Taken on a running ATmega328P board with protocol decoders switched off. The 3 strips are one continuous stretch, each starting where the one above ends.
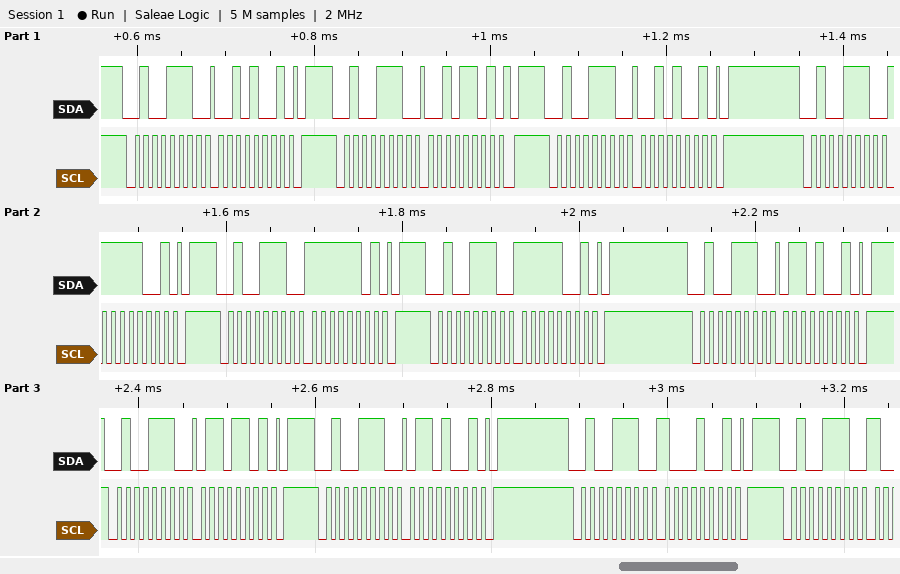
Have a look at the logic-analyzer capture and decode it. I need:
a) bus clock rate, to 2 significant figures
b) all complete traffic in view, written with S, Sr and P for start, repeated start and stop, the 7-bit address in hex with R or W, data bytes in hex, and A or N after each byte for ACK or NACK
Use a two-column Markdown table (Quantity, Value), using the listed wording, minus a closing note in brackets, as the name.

| Quantity | Value |
|---|---|
| bus clock rate, to 2 significant figures | 100 kHz |
| all complete traffic in view, written with S, Sr and P for start, repeated start and stop, the 7-bit address in hex with R or W, data bytes in hex, and A or N after each byte for ACK or NACK | S 27W A 29 A P S 27W A 2D A P S 27W A 29 A P S 27W A F9 A P S 27W A FD A P S 27W A F9 A P S 27W A 69 A P S 27W A 6D A P S 27W A 69 A P S 27W A 89 A P S 27W A |
